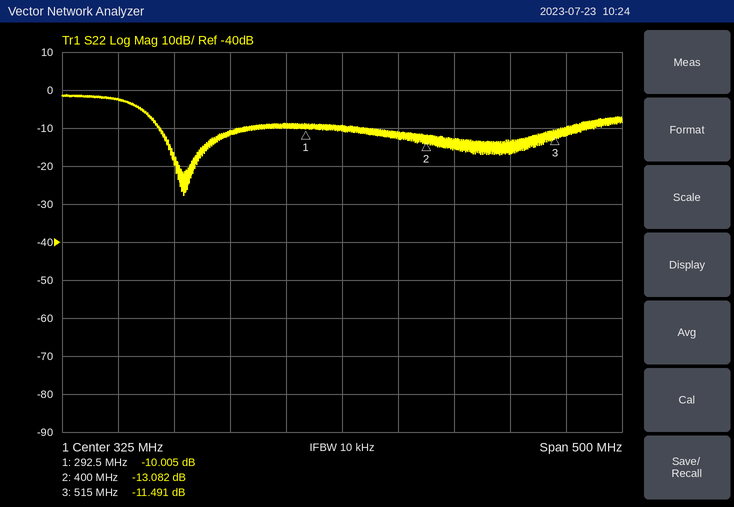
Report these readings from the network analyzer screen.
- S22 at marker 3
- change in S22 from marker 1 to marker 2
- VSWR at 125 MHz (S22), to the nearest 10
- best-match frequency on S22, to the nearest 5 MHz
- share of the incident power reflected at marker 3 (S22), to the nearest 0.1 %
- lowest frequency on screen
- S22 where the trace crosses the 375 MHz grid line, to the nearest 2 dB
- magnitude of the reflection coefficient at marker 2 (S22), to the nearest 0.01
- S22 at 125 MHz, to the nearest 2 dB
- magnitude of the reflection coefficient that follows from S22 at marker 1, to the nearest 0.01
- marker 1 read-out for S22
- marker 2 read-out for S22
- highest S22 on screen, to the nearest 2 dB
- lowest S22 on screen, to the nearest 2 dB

-11.491 dB
-3.077 dB
10
185 MHz
7.1 %
75 MHz
-12 dB
0.22
-2 dB
0.32
-10.005 dB
-13.082 dB
-2 dB
-28 dB
